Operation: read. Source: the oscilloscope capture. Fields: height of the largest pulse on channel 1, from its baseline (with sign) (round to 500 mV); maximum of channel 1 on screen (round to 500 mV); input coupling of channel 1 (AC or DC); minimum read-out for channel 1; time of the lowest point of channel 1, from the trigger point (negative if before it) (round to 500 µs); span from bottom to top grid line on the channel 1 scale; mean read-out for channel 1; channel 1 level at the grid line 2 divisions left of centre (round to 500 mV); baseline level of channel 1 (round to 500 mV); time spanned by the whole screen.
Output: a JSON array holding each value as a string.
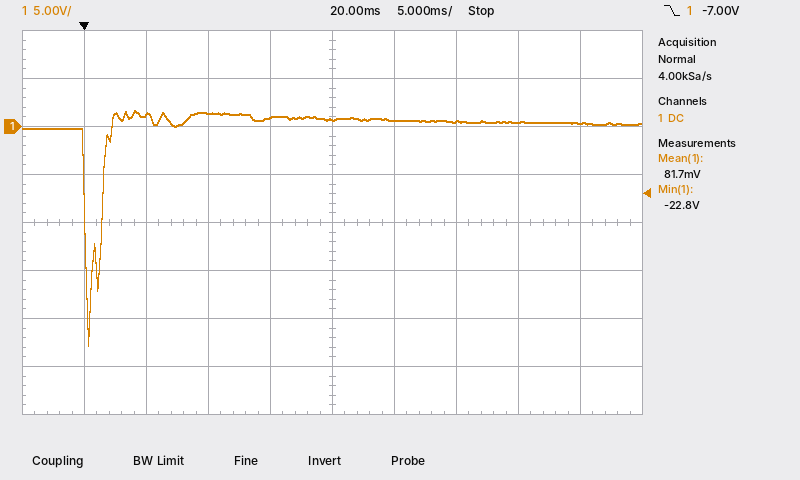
["-23.5 V", "1.5 V", "DC", "-22.8 V", "+500 µs", "40 V", "81.7 mV", "1.5 V", "500 mV", "50 ms"]
